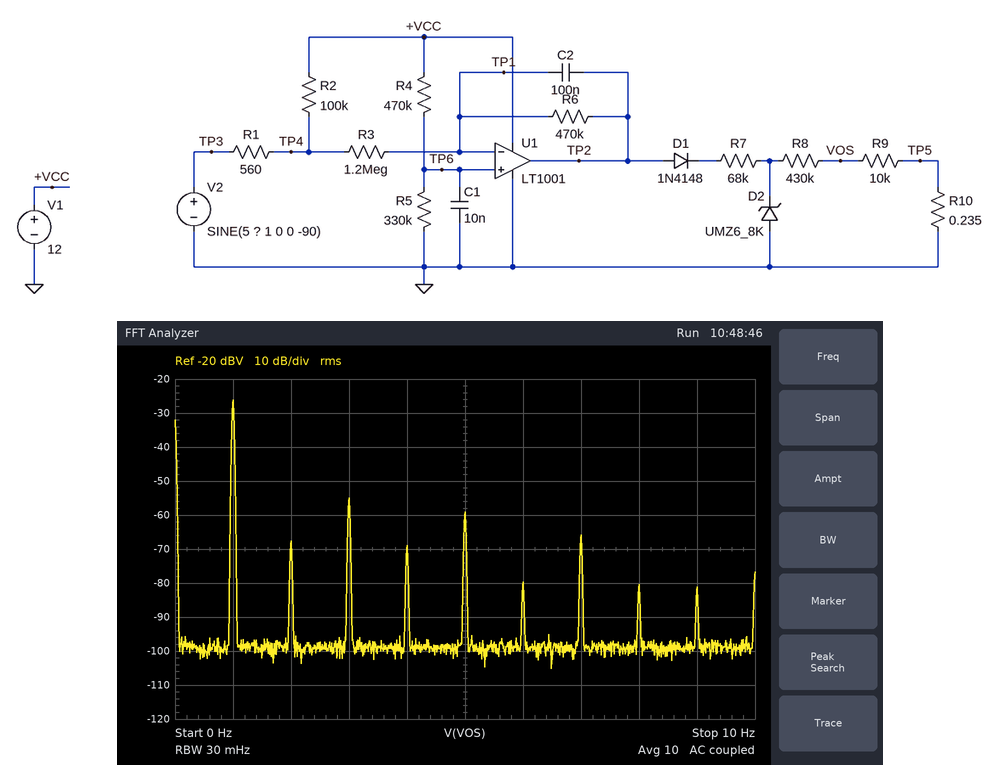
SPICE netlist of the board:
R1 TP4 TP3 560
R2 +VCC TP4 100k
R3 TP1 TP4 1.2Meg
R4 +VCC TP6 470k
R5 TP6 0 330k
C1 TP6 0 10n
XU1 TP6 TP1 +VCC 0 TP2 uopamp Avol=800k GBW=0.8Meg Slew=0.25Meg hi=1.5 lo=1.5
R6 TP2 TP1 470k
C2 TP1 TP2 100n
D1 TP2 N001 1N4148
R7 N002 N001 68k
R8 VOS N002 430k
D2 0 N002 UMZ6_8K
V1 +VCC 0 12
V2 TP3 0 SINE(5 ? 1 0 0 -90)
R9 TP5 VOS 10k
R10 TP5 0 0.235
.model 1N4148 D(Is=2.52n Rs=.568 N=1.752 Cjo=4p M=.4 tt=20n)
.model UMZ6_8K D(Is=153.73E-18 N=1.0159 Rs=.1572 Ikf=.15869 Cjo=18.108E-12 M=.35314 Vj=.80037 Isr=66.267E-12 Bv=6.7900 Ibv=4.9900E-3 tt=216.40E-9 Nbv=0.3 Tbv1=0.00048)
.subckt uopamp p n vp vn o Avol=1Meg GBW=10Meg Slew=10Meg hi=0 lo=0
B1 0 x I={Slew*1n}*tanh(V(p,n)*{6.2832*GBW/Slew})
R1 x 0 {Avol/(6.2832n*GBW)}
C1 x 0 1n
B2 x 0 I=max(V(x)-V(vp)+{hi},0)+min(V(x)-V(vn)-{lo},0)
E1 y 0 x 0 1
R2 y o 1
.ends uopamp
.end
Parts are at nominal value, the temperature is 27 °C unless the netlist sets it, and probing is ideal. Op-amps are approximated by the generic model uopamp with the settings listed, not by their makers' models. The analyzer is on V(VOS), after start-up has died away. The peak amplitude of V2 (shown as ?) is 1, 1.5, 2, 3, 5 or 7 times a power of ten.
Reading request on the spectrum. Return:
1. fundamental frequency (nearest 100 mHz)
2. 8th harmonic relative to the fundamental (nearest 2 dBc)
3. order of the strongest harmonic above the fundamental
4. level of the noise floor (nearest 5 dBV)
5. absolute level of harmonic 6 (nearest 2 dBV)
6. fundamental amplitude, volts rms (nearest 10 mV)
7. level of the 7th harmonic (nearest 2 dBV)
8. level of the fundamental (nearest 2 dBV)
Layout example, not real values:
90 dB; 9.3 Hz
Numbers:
1.0 Hz; -54 dBc; 3; -100 dBV; -80 dBV; 50 mV; -66 dBV; -26 dBV
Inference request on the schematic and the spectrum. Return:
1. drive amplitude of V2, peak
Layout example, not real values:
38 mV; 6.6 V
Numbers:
10 V
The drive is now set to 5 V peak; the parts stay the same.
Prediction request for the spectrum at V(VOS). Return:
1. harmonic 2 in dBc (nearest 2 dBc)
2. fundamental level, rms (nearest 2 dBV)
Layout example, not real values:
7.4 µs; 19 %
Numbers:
-60 dBc; -32 dBV
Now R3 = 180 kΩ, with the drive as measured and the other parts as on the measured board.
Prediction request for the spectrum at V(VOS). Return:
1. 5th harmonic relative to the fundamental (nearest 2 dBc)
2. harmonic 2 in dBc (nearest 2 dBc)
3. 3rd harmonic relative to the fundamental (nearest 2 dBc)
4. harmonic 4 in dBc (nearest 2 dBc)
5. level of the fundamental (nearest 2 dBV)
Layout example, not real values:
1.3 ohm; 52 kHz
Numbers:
-16 dBc; -38 dBc; -10 dBc; -38 dBc; -24 dBV
